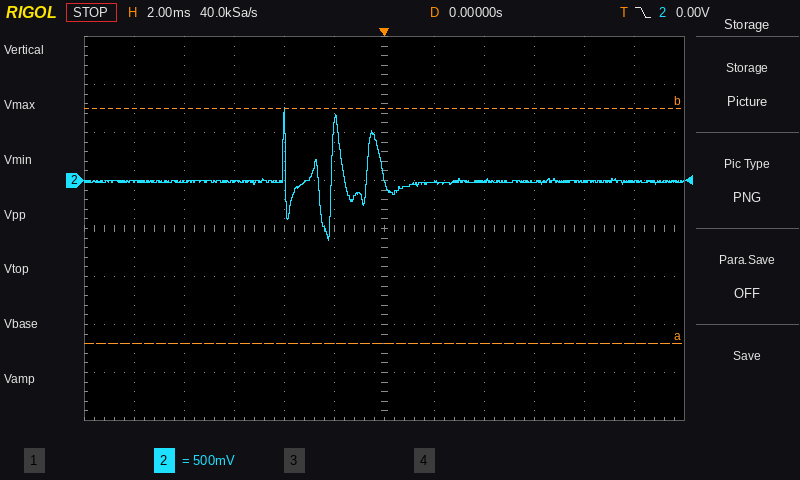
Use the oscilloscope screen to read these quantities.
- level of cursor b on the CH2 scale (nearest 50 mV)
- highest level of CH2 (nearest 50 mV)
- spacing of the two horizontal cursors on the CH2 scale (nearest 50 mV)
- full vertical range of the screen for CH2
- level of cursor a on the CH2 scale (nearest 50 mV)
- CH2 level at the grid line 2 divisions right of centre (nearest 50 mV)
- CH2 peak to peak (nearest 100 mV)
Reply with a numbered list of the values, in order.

1. 750 mV
2. 750 mV
3. 2.45 V
4. 4 V
5. -1.70 V
6. 0 mV
7. 1.40 V
